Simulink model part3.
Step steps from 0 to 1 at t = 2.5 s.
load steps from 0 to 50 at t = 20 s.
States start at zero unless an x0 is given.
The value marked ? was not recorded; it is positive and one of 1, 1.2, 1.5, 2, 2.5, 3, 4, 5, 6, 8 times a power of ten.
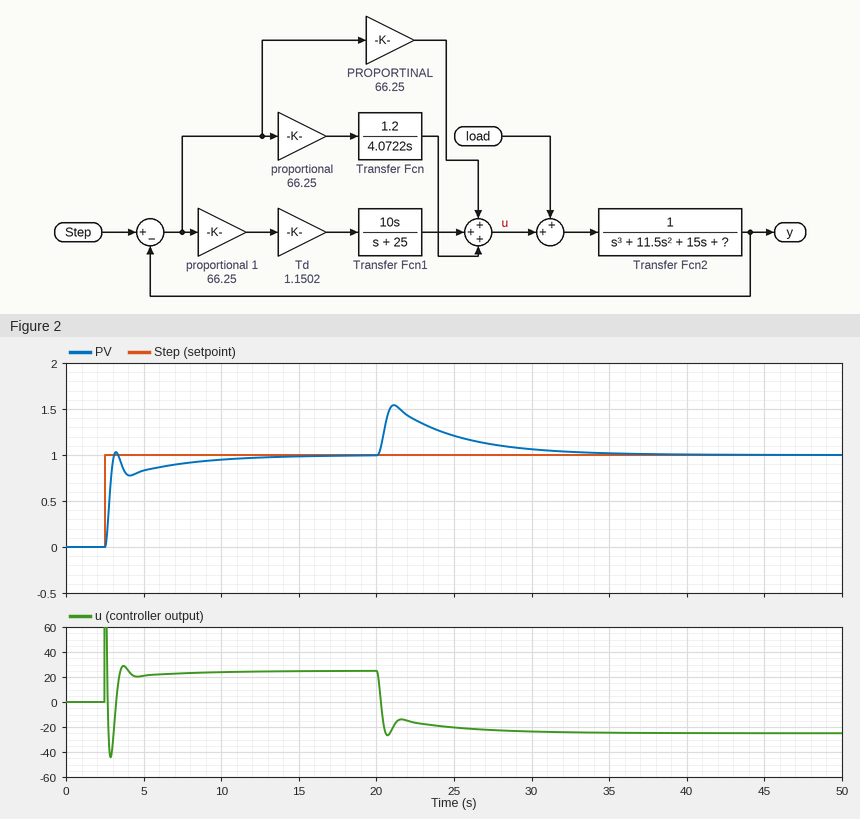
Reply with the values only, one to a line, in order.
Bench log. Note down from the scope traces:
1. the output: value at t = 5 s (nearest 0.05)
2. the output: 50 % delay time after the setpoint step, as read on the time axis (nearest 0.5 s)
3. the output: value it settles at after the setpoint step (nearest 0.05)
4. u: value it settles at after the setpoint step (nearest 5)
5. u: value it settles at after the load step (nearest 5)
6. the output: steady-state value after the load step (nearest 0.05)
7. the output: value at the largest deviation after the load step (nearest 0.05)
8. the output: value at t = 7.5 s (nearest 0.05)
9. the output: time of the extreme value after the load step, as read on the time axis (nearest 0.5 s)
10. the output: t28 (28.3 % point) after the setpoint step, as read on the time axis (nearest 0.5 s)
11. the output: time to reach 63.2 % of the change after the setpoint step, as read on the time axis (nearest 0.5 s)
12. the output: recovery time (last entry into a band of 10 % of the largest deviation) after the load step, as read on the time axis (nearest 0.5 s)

0.85
3.0 s
1.00
25
-25
1.00
1.55
0.90
21.0 s
2.5 s
3.0 s
30.5 s
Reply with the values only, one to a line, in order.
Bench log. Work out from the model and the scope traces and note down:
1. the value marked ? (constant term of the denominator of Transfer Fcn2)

25
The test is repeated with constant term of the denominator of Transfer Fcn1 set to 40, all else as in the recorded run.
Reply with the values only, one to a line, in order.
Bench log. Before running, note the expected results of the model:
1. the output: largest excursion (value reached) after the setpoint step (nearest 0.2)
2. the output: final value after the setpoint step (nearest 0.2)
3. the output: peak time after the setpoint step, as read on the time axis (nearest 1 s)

1.0
1.0
3 s
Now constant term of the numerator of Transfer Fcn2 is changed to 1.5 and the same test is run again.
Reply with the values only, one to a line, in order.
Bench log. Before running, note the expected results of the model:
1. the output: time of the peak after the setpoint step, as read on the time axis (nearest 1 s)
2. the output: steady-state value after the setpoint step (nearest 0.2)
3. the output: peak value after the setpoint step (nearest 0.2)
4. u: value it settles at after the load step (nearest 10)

3 s
1.0
1.2
-30
